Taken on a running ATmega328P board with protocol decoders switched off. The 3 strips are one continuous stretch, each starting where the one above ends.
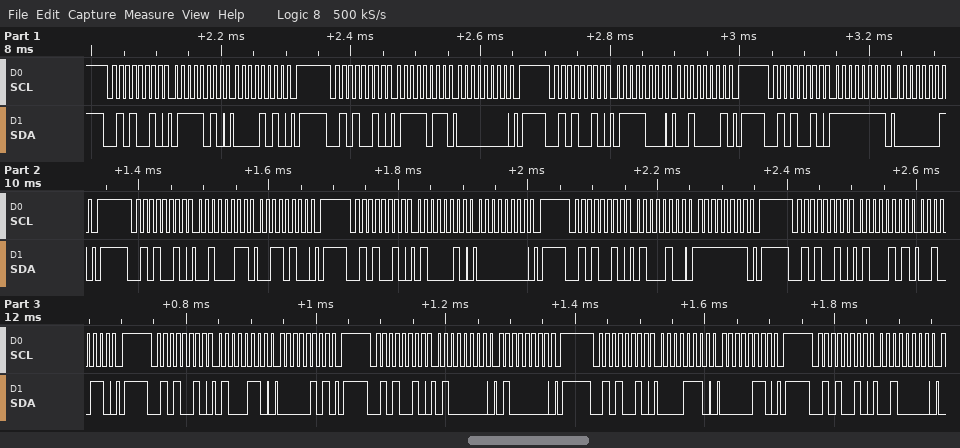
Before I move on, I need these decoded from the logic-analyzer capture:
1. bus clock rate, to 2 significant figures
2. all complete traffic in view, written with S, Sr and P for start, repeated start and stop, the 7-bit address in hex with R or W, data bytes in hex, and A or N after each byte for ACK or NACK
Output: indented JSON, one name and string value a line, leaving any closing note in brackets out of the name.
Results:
{
  "bus clock rate, to 2 significant figures": "100 kHz",
  "all complete traffic in view, written with S, Sr and P for start, repeated start and stop, the 7-bit address in hex with R or W, data bytes in hex, and A or N after each byte for ACK or NACK": "S 29W A 7A A 0A A P S 29W A 7B A 00 A P S 29W A 78 A 21 A P S 29W A FF A 01 A P S 29W A 23 A 34 A P S 29W A 42 A 00 A P S 29W A 44 A FF A P S 29W A 45 A 26 A P S 29W A 46 A 05 A P S 29W A 40 A 40 A P S 29W A 0E A 06 A P S 29W A 20 A"
}
